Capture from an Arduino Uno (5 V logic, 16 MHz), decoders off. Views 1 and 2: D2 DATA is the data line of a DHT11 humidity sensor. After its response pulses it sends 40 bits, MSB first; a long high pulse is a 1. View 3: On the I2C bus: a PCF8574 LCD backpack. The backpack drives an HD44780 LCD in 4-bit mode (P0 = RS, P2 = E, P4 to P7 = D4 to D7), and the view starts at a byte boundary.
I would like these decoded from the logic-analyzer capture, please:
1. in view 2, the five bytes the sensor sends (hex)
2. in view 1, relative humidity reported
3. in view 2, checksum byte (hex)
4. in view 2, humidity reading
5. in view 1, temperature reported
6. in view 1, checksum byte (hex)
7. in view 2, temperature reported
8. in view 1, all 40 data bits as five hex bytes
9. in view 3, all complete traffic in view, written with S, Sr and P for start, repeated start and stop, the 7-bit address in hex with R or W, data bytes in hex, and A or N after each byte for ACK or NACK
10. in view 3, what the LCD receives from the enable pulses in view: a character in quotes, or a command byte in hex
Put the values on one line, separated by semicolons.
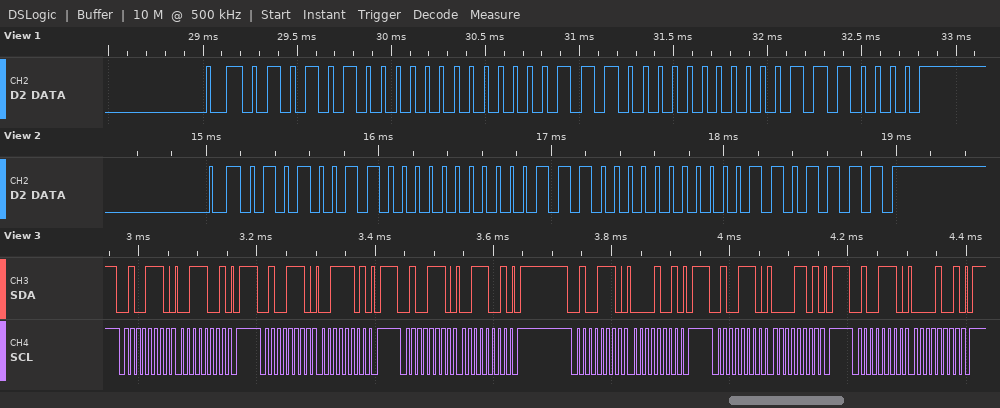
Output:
53 00 1C 00 6F; 84 %; 0x6F; 83 %; 28.0 °C; 0x70; 28.0 °C; 54 00 1C 00 70; S 27W A 39 A P S 27W A 3D A P S 27W A 39 A P S 27W A 09 A P S 27W A 0D A P S 27W A 09 A P; '0'
